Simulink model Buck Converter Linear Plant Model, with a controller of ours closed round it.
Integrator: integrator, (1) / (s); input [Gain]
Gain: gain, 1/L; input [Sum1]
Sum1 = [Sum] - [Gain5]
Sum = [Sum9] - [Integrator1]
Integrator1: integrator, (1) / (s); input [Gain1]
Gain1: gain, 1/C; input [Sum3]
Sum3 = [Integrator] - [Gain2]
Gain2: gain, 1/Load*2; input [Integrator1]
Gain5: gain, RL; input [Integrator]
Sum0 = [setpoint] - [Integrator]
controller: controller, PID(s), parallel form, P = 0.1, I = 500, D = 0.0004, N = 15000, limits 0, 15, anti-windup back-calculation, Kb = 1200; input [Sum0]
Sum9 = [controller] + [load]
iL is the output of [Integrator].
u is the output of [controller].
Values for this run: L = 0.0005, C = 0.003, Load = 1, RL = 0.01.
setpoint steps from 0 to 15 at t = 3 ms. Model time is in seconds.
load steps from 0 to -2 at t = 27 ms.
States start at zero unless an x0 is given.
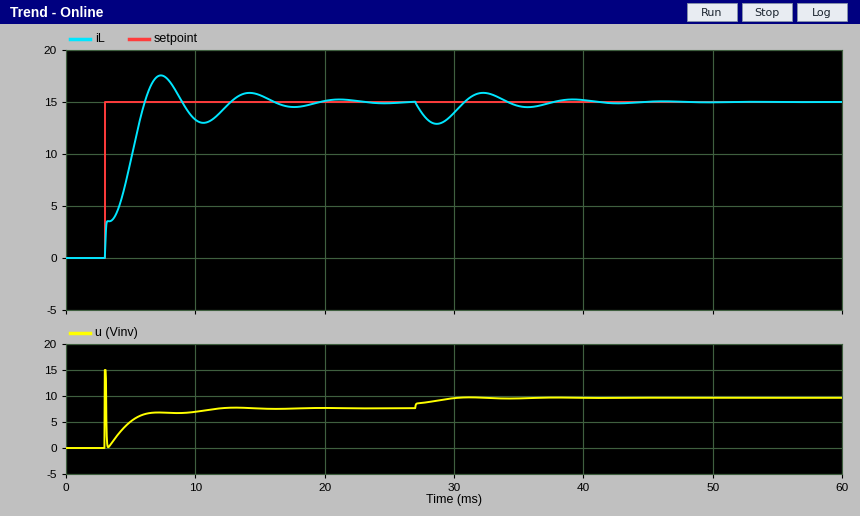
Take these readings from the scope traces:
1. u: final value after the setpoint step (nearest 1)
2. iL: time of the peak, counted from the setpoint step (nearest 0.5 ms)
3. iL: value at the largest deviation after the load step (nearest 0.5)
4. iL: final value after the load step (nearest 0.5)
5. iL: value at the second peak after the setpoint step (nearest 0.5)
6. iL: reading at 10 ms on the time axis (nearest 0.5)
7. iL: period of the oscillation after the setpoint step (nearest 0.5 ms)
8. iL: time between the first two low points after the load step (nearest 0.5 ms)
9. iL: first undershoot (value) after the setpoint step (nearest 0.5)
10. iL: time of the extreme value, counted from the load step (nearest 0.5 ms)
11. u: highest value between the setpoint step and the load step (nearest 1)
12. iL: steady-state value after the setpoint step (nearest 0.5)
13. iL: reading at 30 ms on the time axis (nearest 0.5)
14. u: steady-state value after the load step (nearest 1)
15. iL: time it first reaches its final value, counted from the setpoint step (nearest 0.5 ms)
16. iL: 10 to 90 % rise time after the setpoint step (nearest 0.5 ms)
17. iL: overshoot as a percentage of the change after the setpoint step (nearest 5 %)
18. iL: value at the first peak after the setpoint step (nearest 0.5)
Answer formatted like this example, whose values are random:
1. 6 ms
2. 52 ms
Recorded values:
1. 8
2. 4.5 ms
3. 13.0
4. 15.0
5. 16.0
6. 13.5
7. 7.0 ms
8. 7.0 ms
9. 13.0
10. 1.5 ms
11. 15
12. 15.0
13. 14.0
14. 10
15. 3.0 ms
16. 2.5 ms
17. 15 %
18. 17.5
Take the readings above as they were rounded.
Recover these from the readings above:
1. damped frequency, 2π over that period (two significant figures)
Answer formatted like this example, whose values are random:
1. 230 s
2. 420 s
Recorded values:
1. 0.90 rad/ms
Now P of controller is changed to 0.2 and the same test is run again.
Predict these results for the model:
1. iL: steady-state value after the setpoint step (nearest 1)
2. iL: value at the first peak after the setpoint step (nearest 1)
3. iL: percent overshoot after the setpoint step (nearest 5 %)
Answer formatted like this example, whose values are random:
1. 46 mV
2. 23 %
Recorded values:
1. 15
2. 16
3. 10 %
